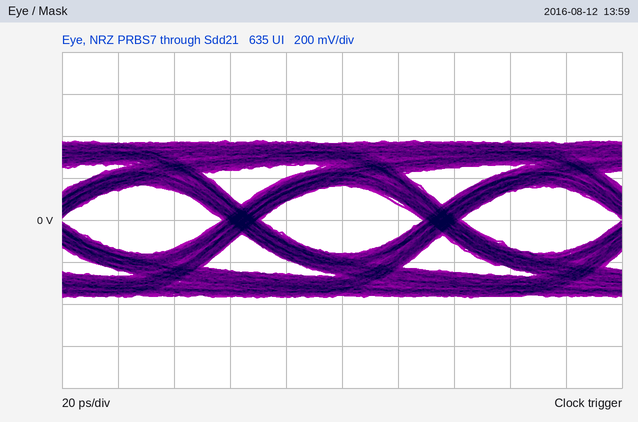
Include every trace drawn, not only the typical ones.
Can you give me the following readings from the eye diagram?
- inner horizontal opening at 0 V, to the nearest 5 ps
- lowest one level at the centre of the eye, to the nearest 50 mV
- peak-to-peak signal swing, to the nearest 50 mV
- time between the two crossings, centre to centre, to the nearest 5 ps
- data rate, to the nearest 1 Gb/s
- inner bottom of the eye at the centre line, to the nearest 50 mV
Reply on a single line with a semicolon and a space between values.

60 ps; 150 mV; 750 mV; 70 ps; 14 Gb/s; -150 mV
